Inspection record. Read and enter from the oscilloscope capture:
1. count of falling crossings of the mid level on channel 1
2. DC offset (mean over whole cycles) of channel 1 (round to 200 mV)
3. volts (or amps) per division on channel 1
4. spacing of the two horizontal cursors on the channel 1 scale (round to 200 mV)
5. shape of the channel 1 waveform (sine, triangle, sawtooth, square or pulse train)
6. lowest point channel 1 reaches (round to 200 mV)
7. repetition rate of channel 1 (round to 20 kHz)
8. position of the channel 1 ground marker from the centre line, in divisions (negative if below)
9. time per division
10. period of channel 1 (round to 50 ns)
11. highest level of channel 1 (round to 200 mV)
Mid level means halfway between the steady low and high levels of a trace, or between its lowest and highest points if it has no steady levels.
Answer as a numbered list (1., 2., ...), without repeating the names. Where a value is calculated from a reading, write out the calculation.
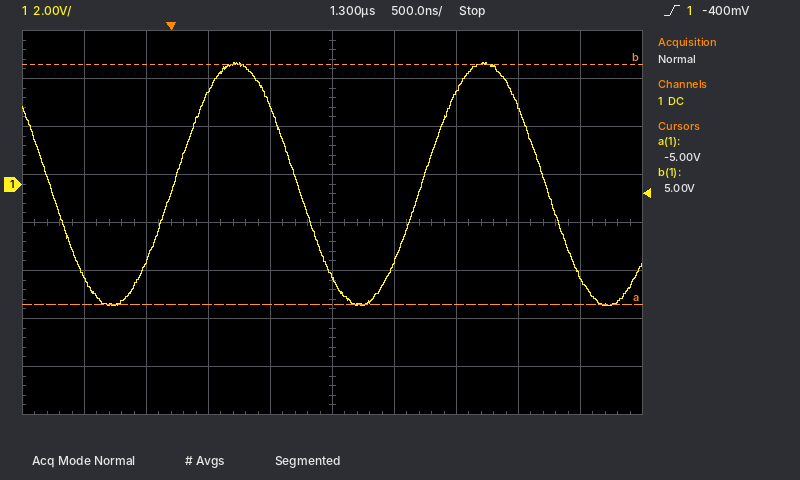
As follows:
1. 3
2. (5.0 V + (-5.0 V)) / 2 ≈ 0.0 V
3. 2 V
4. 10.0 V
5. sine
6. -5.0 V
7. 1 / 2.00 µs ≈ 500 kHz
8. +0.8 div
9. 500 ns
10. 2.00 µs
11. 5.0 V
